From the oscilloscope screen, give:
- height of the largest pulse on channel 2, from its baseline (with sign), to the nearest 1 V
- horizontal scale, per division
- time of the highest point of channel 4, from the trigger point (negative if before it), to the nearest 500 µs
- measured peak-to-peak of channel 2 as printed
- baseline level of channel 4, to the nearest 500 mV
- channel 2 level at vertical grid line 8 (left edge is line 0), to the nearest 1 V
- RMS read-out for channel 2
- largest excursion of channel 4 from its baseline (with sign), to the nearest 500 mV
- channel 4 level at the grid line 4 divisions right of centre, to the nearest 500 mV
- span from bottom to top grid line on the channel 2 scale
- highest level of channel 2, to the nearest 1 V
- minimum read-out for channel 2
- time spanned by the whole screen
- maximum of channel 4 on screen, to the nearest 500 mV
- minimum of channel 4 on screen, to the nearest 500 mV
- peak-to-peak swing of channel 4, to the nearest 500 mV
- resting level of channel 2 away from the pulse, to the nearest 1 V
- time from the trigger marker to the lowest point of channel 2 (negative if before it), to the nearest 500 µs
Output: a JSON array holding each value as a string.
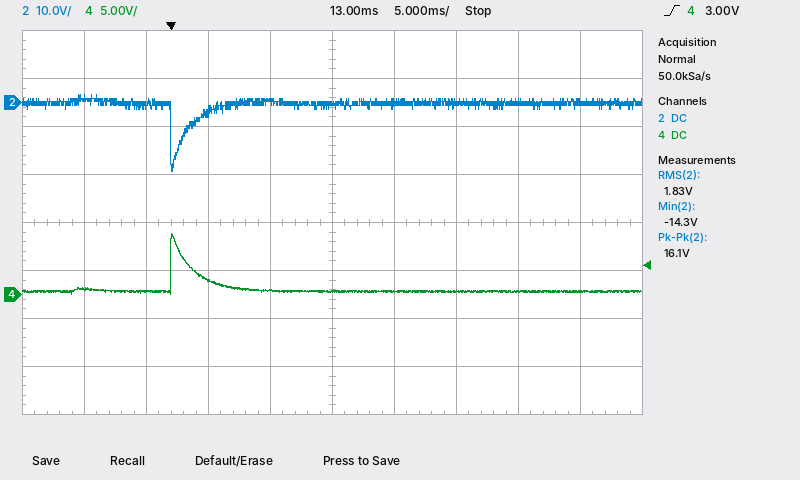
["-14 V", "5 ms", "0.0 ms", "16.1 V", "500 mV", "0 V", "1.83 V", "+6.0 V", "500 mV", "80 V", "2 V", "-14.3 V", "50 ms", "6.5 V", "0.0 V", "6.5 V", "0 V", "0.0 ms"]
